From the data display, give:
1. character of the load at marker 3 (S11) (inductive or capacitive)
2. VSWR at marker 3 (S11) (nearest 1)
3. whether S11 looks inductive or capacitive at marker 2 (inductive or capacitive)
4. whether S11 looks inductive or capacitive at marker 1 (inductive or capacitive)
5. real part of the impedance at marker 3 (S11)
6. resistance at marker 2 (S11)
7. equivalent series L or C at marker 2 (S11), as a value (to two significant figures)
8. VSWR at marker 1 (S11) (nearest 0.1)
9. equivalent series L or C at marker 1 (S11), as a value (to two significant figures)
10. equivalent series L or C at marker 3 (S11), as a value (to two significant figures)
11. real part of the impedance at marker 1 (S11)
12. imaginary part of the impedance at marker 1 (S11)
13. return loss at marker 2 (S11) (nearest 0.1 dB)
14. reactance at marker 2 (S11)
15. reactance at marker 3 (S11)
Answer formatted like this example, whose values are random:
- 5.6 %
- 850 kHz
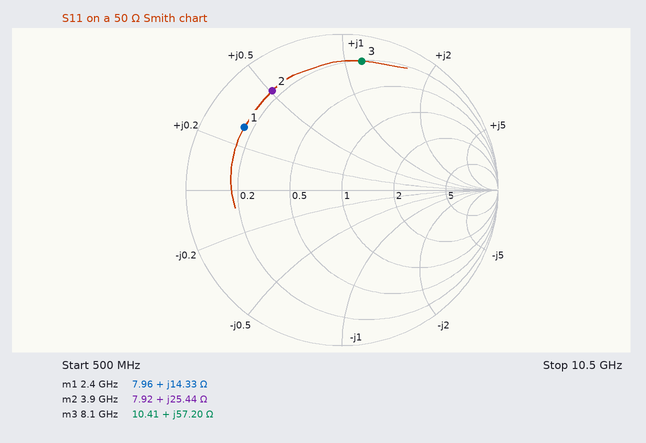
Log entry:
- inductive
- 11
- inductive
- inductive
- 10.41 Ω
- 7.92 Ω
- 1.0 nH
- 6.8
- 950 pH
- 1.1 nH
- 7.96 Ω
- +14.33 Ω
- 2.2 dB
- +25.44 Ω
- +57.20 Ω
